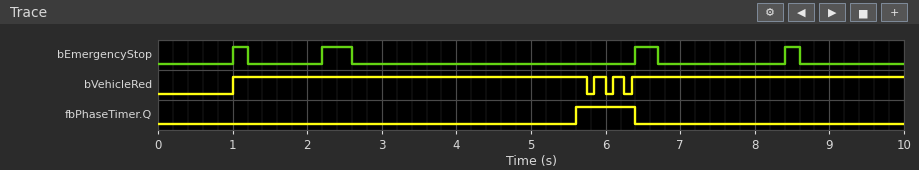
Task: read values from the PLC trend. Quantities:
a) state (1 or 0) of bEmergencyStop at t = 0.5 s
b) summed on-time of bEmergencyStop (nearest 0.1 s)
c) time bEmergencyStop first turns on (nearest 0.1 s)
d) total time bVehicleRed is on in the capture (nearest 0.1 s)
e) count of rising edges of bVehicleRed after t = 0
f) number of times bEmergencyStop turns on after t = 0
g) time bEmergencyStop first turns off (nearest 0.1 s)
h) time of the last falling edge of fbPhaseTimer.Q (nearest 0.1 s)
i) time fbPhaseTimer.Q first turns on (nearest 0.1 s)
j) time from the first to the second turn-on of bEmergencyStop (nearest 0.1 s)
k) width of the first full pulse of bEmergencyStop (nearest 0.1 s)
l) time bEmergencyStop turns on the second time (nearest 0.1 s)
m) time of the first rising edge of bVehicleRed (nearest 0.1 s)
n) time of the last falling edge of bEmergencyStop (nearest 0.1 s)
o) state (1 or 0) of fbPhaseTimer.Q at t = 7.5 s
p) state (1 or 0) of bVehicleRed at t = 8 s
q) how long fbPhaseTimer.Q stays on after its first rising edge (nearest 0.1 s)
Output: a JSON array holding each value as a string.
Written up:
["0", "1.1 s", "1.0 s", "8.7 s", "4", "4", "1.2 s", "6.4 s", "5.6 s", "1.2 s", "0.2 s", "2.2 s", "1.0 s", "8.6 s", "0", "1", "0.8 s"]
